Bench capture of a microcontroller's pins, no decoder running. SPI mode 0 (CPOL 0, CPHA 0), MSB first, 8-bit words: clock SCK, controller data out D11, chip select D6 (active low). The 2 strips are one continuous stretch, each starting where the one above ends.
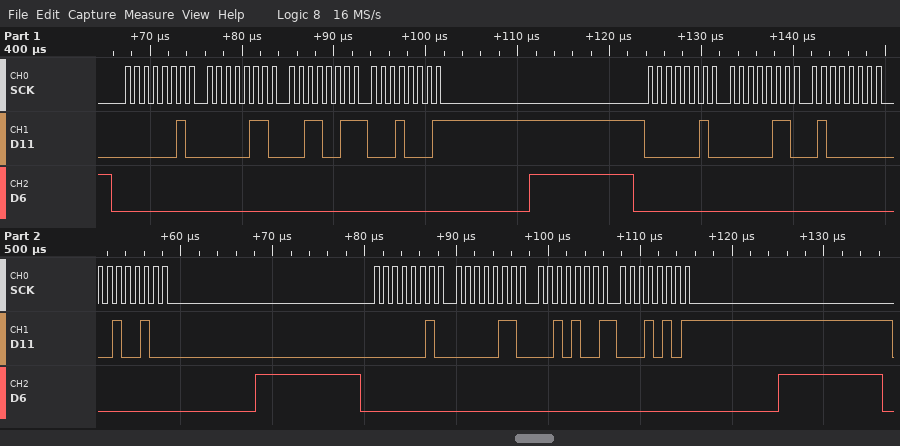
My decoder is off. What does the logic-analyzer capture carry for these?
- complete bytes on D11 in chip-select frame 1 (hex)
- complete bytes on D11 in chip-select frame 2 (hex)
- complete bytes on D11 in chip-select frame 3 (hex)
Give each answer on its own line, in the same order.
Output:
02 06 33 11
02 06 40 24
02 06 29 15
